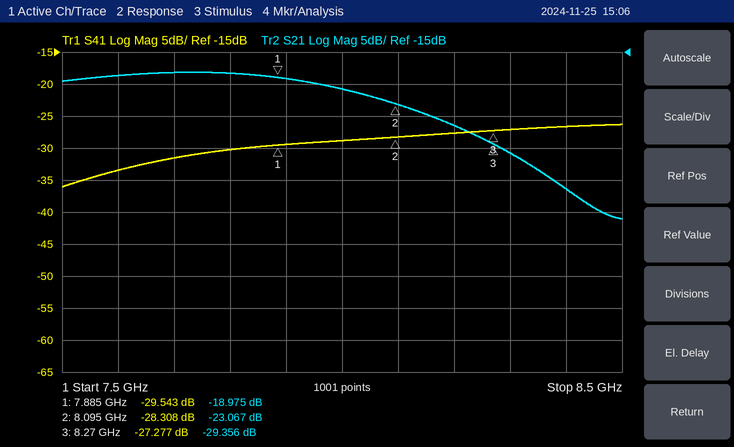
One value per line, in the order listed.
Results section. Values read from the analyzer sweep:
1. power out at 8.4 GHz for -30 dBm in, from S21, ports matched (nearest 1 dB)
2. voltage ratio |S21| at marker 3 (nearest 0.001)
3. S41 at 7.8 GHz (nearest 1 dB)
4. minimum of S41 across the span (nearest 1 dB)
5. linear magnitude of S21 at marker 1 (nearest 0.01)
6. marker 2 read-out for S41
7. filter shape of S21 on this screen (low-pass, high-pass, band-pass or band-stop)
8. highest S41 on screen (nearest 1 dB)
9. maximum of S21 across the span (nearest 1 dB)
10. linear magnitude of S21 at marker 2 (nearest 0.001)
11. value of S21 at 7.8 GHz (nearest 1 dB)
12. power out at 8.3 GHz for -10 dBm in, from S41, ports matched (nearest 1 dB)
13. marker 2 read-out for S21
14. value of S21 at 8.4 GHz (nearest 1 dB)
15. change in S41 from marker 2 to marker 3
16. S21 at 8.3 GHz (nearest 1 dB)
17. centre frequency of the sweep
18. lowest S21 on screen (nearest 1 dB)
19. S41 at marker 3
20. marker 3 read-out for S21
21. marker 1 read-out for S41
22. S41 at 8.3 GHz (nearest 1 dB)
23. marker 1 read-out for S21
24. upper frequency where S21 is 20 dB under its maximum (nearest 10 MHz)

-66 dBm
0.034
-30 dB
-36 dB
0.11
-28.308 dB
low-pass
-26 dB
-18 dB
0.070
-18 dB
-37 dBm
-23.067 dB
-36 dB
1.031 dB
-31 dB
8 GHz
-41 dB
-27.277 dB
-29.356 dB
-29.543 dB
-27 dB
-18.975 dB
8.43 GHz
